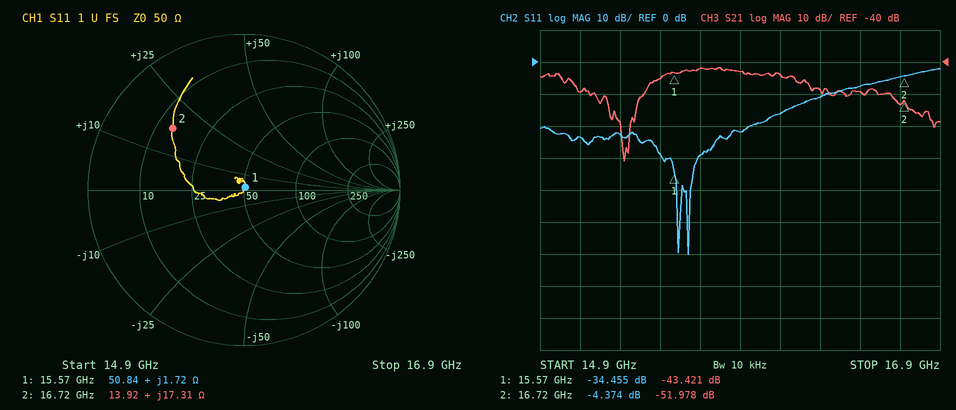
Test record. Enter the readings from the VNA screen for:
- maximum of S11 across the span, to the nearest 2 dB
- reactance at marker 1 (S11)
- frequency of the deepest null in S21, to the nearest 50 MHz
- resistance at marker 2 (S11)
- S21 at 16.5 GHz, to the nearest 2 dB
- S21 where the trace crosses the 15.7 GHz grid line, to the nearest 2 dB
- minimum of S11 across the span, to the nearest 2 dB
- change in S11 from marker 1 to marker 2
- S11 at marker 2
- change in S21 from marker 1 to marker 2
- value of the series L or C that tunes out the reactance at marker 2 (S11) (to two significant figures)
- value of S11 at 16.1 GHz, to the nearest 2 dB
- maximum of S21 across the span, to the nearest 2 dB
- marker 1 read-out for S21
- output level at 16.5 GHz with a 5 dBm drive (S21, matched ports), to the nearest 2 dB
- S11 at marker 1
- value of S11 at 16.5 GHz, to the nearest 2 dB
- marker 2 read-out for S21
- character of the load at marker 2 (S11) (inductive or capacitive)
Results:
-2 dB
+1.72 Ω
15.30 GHz
13.92 Ω
-50 dB
-42 dB
-60 dB
30.081 dB
-4.374 dB
-8.557 dB
550 fF
-16 dB
-42 dB
-43.421 dB
-44 dBm
-34.455 dB
-8 dB
-51.978 dB
inductive
